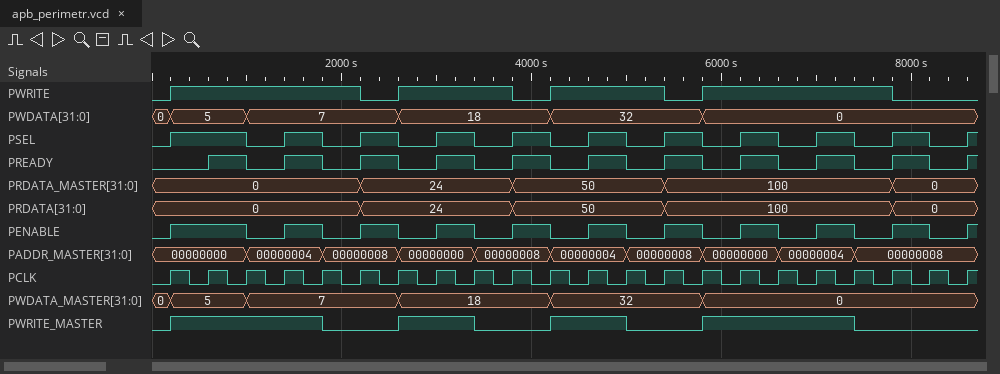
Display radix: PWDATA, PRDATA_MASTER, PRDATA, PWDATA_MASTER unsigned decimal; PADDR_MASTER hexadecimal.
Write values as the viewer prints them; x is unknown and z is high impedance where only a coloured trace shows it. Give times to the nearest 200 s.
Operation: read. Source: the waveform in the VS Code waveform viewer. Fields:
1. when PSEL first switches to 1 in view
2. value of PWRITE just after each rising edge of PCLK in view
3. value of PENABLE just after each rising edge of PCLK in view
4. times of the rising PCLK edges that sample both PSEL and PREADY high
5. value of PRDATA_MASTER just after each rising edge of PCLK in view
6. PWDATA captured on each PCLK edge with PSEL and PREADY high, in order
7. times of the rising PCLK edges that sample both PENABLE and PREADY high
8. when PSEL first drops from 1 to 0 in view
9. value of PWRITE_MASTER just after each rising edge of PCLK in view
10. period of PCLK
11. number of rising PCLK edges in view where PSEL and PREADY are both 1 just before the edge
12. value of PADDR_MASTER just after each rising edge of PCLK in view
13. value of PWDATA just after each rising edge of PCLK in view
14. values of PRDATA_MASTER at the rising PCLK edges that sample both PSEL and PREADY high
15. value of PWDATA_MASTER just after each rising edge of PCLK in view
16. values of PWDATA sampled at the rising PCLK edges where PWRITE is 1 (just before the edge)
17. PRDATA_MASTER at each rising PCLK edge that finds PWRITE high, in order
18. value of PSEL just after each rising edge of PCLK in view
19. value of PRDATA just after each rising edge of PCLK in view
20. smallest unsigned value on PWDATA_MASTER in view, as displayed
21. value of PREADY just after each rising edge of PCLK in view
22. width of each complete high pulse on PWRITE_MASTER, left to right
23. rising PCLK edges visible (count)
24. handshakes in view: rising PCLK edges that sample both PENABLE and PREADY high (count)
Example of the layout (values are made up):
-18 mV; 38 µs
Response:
200 s; 1 1 1 1 1 0 1 1 1 0 1 1 1 0 1 1 1 1 1 0 0 0; 1 1 0 1 0 1 0 1 0 1 0 1 0 1 0 1 0 1 0 1 0 1; 1000 s, 1800 s, 2600 s, 3400 s, 4200 s, 5000 s, 5800 s, 6600 s, 7400 s, 8200 s; 0, 0, 0, 0, 0, 24, 24, 24, 24, 50, 50, 50, 50, 100, 100, 100, 100, 100, 100, 0, 0, 0; 5, 7, 7, 18, 18, 32, 32, 0, 0, 0; 1000 s, 1800 s, 2600 s, 3400 s, 4200 s, 5000 s, 5800 s, 6600 s, 7400 s, 8200 s; 1000 s; 1 1 1 1 0 0 1 1 0 0 1 1 0 0 1 1 1 1 0 0 0 0; 400 s; 10; 00000000, 00000000, 00000004, 00000004, 00000008, 00000008, 00000000, 00000000, 00000008, 00000008, 00000004, 00000004, 00000008, 00000008, 00000000, 00000000, 00000004, 00000004, 00000008, 00000008, 00000008, 00000008; 5, 5, 7, 7, 7, 7, 18, 18, 18, 18, 32, 32, 32, 32, 0, 0, 0, 0, 0, 0, 0, 0; 0, 0, 24, 24, 50, 50, 100, 100, 100, 0; 5, 5, 7, 7, 7, 7, 18, 18, 18, 18, 32, 32, 32, 32, 0, 0, 0, 0, 0, 0, 0, 0; 5, 5, 7, 7, 7, 18, 18, 18, 32, 32, 32, 0, 0, 0, 0, 0; 0, 0, 0, 0, 0, 24, 24, 24, 50, 50, 50, 100, 100, 100, 100, 100; 1 1 0 1 0 1 0 1 0 1 0 1 0 1 0 1 0 1 0 1 0 1; 0, 0, 0, 0, 0, 24, 24, 24, 24, 50, 50, 50, 50, 100, 100, 100, 100, 100, 100, 0, 0, 0; 0; 0 1 0 1 0 1 0 1 0 1 0 1 0 1 0 1 0 1 0 1 0 1; 1600 s, 800 s, 800 s, 1600 s; 22; 10
